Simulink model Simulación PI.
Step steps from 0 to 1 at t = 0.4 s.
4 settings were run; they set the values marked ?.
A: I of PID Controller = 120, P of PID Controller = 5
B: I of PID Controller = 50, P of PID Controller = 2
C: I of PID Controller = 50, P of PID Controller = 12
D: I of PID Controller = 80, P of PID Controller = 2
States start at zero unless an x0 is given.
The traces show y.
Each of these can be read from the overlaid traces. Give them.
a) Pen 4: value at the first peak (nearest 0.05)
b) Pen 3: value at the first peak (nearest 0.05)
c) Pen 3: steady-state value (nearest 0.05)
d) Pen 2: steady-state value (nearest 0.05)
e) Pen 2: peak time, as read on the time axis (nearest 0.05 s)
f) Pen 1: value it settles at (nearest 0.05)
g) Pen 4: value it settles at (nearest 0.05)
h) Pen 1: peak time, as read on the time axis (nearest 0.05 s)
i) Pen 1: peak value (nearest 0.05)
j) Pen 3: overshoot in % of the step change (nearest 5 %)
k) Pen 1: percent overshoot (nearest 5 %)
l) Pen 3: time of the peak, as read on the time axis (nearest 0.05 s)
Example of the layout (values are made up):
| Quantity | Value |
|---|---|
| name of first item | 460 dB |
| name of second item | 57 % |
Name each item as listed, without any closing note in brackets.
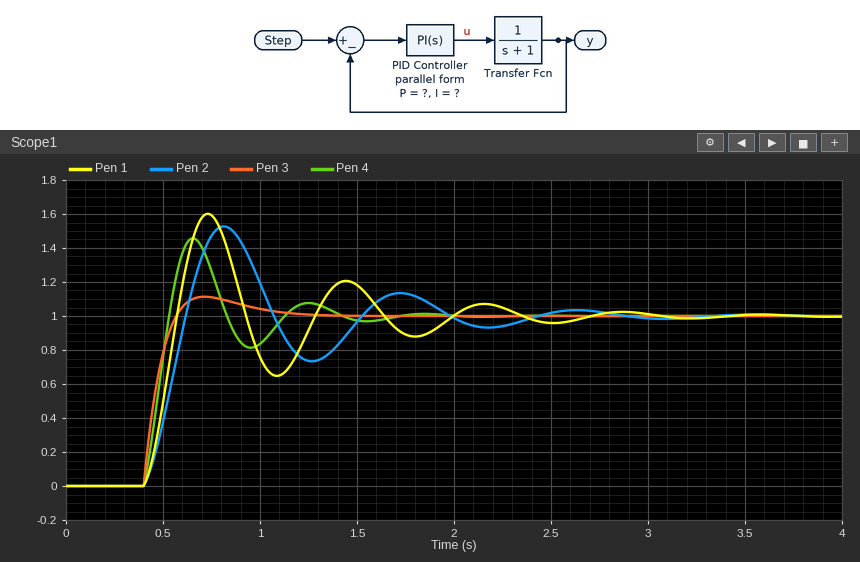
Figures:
| Quantity | Value |
|---|---|
| Pen 4: value at the first peak | 1.45 |
| Pen 3: value at the first peak | 1.10 |
| Pen 3: steady-state value | 1.00 |
| Pen 2: steady-state value | 1.00 |
| Pen 2: peak time, as read on the time axis | 0.80 s |
| Pen 1: value it settles at | 1.00 |
| Pen 4: value it settles at | 1.00 |
| Pen 1: peak time, as read on the time axis | 0.75 s |
| Pen 1: peak value | 1.60 |
| Pen 3: overshoot in % of the step change | 10 % |
| Pen 1: percent overshoot | 60 % |
| Pen 3: time of the peak, as read on the time axis | 0.70 s |
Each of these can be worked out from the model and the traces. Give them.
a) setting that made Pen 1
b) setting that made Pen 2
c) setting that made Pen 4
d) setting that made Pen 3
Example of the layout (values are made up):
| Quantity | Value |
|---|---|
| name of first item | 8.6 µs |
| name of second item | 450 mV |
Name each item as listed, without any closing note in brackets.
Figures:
| Quantity | Value |
|---|---|
| setting that made Pen 1 | D |
| setting that made Pen 2 | B |
| setting that made Pen 4 | A |
| setting that made Pen 3 | C |
